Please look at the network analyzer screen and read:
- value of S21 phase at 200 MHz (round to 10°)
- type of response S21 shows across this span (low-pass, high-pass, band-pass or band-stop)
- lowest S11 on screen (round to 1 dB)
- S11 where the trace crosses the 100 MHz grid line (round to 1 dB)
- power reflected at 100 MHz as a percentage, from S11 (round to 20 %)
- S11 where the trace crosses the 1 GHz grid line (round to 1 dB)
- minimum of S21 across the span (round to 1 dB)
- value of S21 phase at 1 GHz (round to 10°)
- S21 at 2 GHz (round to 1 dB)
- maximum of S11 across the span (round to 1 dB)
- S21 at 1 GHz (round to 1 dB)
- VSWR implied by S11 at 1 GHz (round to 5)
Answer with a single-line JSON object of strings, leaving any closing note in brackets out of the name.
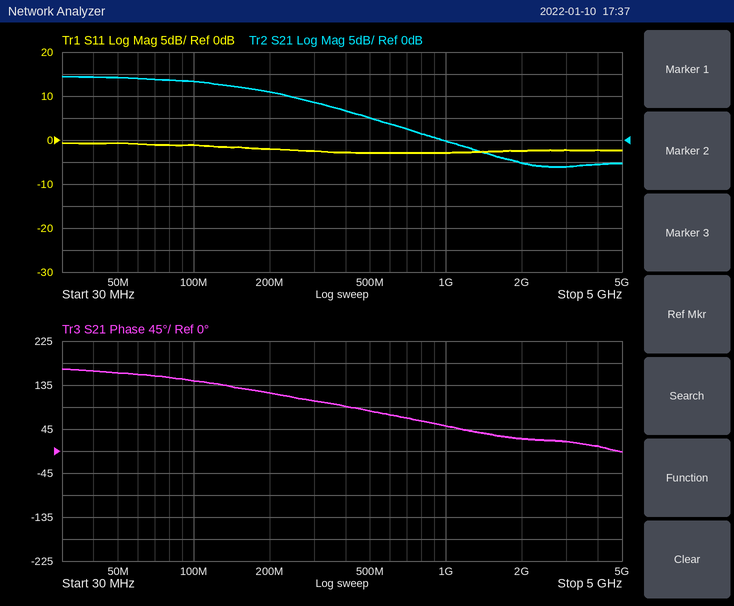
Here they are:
{"value of S21 phase at 200 MHz": "120°", "type of response S21 shows across this span": "low-pass", "lowest S11 on screen": "-3 dB", "S11 where the trace crosses the 100 MHz grid line": "-1 dB", "power reflected at 100 MHz as a percentage, from S11": "80 %", "S11 where the trace crosses the 1 GHz grid line": "-3 dB", "minimum of S21 across the span": "-6 dB", "value of S21 phase at 1 GHz": "50°", "S21 at 2 GHz": "-5 dB", "maximum of S11 across the span": "-1 dB", "S21 at 1 GHz": "0 dB", "VSWR implied by S11 at 1 GHz": "5"}
